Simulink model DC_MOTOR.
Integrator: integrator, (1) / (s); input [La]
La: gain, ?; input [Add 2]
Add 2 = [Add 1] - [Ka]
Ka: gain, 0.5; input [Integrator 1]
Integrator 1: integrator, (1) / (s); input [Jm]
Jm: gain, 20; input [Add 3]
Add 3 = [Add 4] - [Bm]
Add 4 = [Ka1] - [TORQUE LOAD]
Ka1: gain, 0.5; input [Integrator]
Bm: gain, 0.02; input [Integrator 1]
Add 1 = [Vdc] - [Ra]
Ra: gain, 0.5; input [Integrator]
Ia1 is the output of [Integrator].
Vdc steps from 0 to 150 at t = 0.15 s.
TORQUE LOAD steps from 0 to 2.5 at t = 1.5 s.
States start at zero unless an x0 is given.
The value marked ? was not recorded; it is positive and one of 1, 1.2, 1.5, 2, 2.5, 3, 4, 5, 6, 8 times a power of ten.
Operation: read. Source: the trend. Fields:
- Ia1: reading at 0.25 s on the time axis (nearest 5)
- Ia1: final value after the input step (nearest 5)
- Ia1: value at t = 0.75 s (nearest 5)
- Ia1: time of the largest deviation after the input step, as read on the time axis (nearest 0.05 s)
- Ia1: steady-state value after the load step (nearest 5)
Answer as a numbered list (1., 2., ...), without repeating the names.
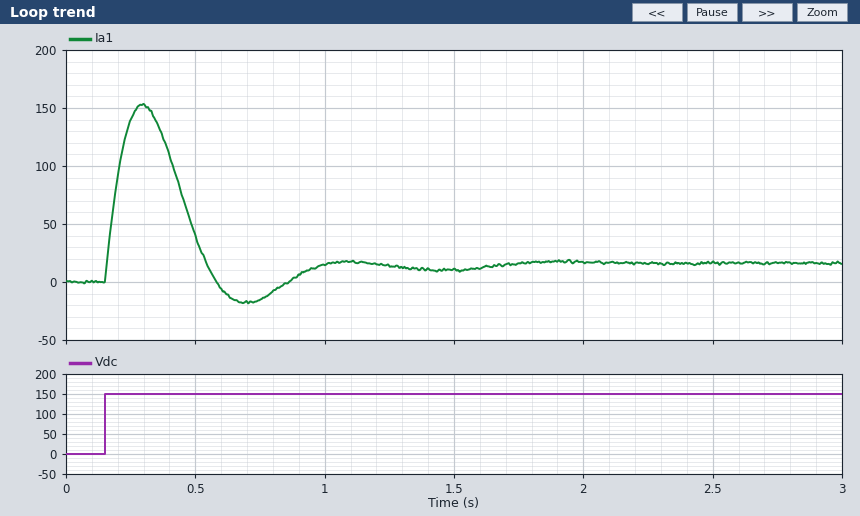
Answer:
1. 140
2. 10
3. -15
4. 0.30 s
5. 15
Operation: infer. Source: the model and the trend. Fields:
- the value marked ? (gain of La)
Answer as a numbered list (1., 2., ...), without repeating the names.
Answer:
1. 15
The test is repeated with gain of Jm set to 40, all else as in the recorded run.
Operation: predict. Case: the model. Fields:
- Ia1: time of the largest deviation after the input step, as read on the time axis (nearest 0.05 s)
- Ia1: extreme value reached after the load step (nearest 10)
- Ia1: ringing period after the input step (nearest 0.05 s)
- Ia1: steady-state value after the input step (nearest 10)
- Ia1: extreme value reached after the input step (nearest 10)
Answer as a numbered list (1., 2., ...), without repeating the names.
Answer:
1. 0.25 s
2. 20
3. 0.55 s
4. 10
5. 120
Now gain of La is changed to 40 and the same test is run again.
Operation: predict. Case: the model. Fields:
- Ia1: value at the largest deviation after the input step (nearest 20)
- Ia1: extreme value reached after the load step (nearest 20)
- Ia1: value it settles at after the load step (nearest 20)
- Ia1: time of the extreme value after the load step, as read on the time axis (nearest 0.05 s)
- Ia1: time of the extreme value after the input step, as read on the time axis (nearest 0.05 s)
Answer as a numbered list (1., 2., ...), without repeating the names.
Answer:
1. 200
2. 20
3. 20
4. 1.80 s
5. 0.25 s
